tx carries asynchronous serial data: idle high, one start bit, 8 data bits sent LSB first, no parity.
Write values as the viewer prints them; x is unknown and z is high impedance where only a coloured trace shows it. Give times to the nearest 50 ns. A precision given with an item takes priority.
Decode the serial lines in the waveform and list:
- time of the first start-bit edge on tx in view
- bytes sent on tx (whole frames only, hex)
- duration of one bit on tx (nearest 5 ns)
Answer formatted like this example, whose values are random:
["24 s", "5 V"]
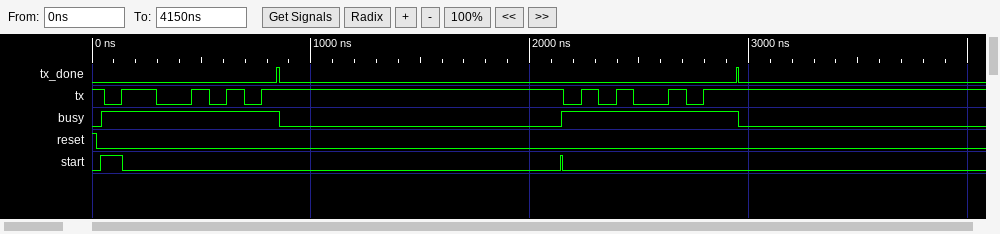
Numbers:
["50 ns", "53, A5", "80 ns"]
